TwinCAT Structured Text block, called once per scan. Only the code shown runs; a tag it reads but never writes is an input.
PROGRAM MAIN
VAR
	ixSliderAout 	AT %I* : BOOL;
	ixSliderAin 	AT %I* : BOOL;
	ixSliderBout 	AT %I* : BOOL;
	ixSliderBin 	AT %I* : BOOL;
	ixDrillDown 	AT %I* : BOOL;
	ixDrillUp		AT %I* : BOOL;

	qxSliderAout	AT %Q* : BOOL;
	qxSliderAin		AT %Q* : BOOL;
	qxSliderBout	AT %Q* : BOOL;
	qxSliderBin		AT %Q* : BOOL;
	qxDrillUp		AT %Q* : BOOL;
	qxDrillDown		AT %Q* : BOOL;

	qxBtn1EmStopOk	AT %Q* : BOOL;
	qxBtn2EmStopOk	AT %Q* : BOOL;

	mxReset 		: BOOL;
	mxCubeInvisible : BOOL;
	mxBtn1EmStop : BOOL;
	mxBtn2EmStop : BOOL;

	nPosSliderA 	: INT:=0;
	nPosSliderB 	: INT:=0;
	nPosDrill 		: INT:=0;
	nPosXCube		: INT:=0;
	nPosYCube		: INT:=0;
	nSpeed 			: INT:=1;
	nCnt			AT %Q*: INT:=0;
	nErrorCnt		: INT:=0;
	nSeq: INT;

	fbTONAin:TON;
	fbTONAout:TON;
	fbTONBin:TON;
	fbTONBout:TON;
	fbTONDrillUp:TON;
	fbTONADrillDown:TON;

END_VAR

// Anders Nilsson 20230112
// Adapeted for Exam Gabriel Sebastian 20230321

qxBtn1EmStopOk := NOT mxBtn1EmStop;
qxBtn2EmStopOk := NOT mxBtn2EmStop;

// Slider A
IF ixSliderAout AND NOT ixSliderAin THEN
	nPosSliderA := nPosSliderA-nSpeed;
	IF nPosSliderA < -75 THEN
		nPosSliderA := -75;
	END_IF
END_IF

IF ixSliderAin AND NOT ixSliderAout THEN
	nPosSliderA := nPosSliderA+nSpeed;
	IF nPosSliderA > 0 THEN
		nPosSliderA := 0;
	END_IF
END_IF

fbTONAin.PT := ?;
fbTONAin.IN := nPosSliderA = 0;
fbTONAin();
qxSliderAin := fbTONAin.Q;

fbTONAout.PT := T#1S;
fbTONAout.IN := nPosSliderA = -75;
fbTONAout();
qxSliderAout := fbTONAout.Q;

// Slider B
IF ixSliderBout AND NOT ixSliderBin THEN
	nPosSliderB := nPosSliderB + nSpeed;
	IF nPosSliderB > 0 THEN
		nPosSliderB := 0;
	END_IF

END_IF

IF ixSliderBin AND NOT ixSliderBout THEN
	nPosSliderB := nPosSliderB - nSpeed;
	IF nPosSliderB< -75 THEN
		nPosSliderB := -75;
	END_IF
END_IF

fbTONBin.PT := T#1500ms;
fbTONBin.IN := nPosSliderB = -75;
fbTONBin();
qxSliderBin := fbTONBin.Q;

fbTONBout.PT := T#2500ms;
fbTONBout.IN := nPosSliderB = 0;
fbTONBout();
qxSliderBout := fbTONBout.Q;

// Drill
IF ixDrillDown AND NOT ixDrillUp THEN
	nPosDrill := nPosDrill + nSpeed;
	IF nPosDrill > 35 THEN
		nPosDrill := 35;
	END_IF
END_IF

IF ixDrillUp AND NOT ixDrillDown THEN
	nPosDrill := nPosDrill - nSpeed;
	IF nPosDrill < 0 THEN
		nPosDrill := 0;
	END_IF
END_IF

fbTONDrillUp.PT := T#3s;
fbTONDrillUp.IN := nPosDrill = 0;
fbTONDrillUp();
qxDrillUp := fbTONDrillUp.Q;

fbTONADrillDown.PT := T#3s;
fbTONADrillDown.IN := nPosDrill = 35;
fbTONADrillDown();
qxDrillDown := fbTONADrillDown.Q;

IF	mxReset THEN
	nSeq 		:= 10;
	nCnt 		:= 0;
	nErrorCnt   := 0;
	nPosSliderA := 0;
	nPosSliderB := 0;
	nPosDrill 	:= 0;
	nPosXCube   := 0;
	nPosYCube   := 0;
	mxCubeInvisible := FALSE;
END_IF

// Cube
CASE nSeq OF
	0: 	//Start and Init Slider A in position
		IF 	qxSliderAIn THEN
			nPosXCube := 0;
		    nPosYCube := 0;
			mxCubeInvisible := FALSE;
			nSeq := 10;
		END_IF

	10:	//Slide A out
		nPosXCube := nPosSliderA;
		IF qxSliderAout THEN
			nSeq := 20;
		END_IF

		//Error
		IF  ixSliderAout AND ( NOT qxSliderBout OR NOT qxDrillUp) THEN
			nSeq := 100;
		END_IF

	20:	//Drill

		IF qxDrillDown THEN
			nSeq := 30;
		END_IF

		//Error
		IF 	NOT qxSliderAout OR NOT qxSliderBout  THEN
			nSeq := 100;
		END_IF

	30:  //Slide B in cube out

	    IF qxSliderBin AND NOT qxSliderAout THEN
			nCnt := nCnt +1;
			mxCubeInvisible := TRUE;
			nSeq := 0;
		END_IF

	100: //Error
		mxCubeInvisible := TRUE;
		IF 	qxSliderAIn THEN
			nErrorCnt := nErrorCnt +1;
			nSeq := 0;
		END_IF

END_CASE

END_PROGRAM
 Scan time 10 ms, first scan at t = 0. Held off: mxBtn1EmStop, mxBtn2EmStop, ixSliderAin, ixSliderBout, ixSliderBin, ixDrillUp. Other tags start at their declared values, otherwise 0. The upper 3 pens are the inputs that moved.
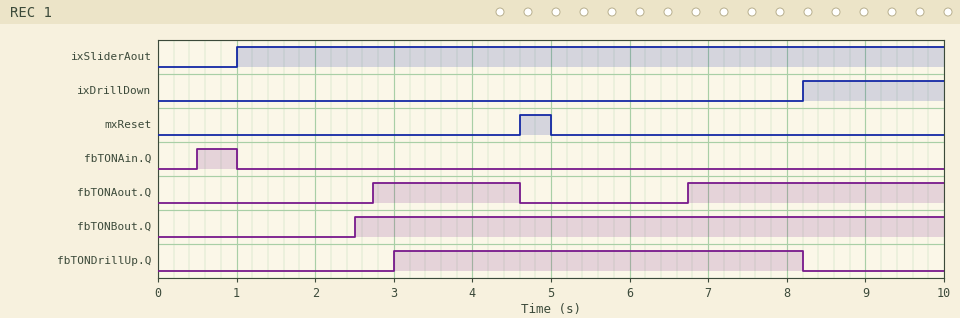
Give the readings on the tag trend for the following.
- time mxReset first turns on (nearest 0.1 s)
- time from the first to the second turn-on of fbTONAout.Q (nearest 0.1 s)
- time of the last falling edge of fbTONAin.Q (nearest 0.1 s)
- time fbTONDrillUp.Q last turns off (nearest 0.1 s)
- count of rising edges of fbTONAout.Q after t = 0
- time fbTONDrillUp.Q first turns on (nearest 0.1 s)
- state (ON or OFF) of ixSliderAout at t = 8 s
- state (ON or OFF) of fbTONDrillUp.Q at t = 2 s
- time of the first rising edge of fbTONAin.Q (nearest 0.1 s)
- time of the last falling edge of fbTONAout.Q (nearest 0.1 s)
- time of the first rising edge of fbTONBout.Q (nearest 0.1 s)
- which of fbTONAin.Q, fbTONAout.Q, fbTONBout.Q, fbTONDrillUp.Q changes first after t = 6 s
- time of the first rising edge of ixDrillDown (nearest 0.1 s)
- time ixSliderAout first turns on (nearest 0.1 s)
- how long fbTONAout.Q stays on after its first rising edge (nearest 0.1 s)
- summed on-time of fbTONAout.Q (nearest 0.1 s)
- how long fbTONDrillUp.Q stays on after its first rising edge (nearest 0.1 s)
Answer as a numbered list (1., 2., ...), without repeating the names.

1. 4.6 s
2. 4.0 s
3. 1.0 s
4. 8.2 s
5. 2
6. 3.0 s
7. ON
8. OFF
9. 0.5 s
10. 4.6 s
11. 2.5 s
12. fbTONAout.Q
13. 8.2 s
14. 1.0 s
15. 1.9 s
16. 5.1 s
17. 5.2 s
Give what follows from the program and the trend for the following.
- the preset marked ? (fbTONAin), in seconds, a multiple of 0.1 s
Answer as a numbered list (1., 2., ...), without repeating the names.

1. 0.5 s
